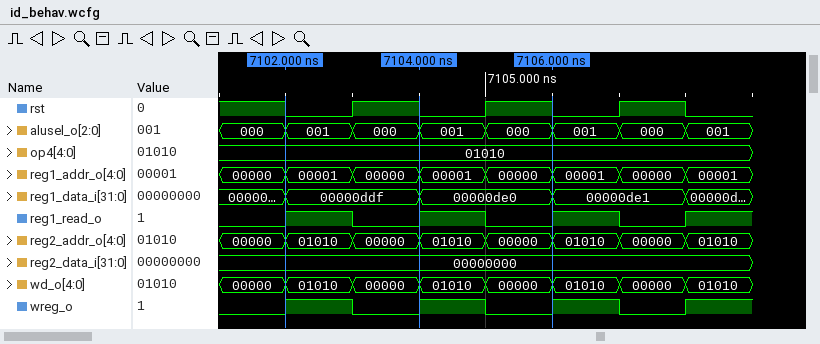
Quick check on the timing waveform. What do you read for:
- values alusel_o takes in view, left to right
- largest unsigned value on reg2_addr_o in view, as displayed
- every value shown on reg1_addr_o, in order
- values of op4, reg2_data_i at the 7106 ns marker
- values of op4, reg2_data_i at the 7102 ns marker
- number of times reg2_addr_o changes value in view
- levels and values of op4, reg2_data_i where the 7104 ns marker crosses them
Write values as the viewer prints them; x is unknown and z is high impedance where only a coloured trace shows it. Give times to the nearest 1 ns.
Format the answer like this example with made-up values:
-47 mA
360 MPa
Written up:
000, 001, 000, 001, 000, 001, 000, 001
01010
00000, 00001, 00000, 00001, 00000, 00001, 00000, 00001
op4=01010, reg2_data_i=00000000
op4=01010, reg2_data_i=00000000
7
op4=01010, reg2_data_i=00000000
